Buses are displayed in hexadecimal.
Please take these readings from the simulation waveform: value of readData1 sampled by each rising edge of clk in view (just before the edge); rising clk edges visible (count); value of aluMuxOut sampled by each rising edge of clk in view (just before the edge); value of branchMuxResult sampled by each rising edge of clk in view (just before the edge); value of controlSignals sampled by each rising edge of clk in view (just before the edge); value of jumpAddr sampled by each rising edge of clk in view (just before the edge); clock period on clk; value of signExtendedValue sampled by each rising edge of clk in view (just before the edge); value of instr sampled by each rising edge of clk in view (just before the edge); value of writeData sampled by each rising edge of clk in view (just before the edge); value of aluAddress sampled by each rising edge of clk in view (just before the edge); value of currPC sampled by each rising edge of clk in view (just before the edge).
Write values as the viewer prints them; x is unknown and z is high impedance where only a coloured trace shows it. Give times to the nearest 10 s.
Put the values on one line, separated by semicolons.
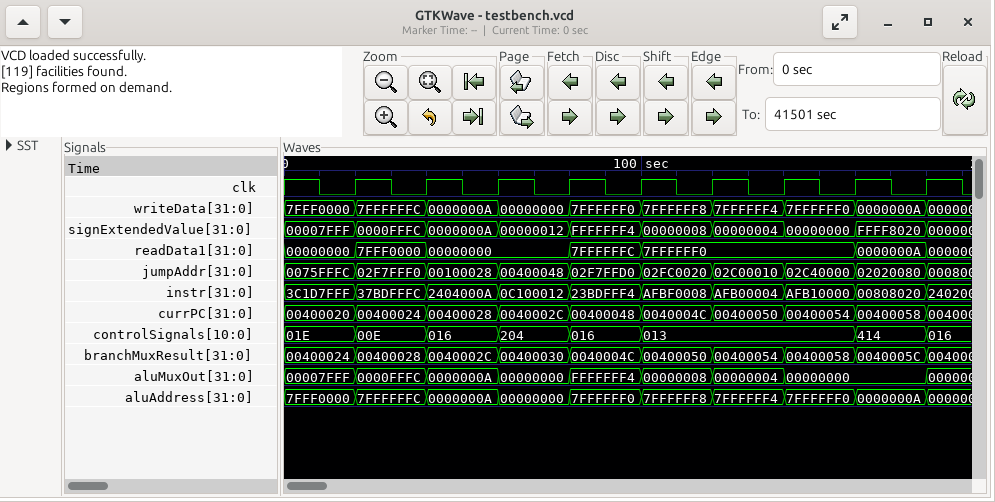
00000000, 7FFF0000, 00000000, 00000000, 7FFFFFFC, 7FFFFFF0, 7FFFFFF0, 7FFFFFF0, 0000000A; 9; 00007FFF, 0000FFFC, 0000000A, 00000000, FFFFFFF4, 00000008, 00000004, 00000000, 00000000; 00400024, 00400028, 0040002C, 00400030, 0040004C, 00400050, 00400054, 00400058, 0040005C; 01E, 00E, 016, 204, 016, 013, 013, 013, 414; 0075FFFC, 02F7FFF0, 00100028, 00400048, 02F7FFD0, 02FC0020, 02C00010, 02C40000, 02020080; 20 s; 00007FFF, 0000FFFC, 0000000A, 00000012, FFFFFFF4, 00000008, 00000004, 00000000, FFFF8020; 3C1D7FFF, 37BDFFFC, 2404000A, 0C100012, 23BDFFF4, AFBF0008, AFB00004, AFB10000, 00808020; 7FFF0000, 7FFFFFFC, 0000000A, 00000000, 7FFFFFF0, 7FFFFFF8, 7FFFFFF4, 7FFFFFF0, 0000000A; 7FFF0000, 7FFFFFFC, 0000000A, 00000000, 7FFFFFF0, 7FFFFFF8, 7FFFFFF4, 7FFFFFF0, 0000000A; 00400020, 00400024, 00400028, 0040002C, 00400048, 0040004C, 00400050, 00400054, 00400058
